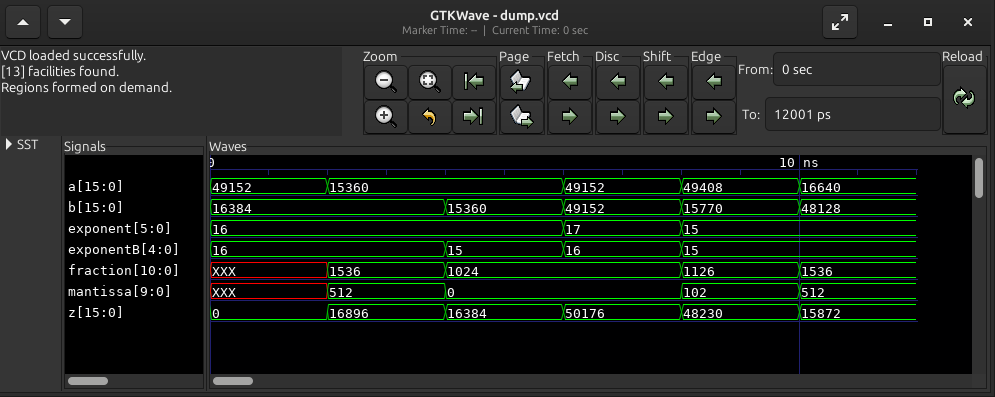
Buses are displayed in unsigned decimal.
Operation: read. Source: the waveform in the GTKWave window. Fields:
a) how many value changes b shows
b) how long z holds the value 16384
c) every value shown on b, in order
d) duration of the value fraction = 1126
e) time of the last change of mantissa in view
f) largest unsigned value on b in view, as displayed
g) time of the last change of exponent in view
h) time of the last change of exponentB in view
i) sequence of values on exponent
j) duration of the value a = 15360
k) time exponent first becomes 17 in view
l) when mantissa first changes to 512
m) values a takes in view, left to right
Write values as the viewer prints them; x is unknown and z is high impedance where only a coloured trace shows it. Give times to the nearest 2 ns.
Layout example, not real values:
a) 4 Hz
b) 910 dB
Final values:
a) 4
b) 2 ns
c) 16384, 15360, 49152, 15770, 48128
d) 2 ns
e) 10 ns
f) 49152
g) 8 ns
h) 8 ns
i) 16, 17, 15
j) 4 ns
k) 6 ns
l) 2 ns
m) 49152, 15360, 49152, 49408, 16640
